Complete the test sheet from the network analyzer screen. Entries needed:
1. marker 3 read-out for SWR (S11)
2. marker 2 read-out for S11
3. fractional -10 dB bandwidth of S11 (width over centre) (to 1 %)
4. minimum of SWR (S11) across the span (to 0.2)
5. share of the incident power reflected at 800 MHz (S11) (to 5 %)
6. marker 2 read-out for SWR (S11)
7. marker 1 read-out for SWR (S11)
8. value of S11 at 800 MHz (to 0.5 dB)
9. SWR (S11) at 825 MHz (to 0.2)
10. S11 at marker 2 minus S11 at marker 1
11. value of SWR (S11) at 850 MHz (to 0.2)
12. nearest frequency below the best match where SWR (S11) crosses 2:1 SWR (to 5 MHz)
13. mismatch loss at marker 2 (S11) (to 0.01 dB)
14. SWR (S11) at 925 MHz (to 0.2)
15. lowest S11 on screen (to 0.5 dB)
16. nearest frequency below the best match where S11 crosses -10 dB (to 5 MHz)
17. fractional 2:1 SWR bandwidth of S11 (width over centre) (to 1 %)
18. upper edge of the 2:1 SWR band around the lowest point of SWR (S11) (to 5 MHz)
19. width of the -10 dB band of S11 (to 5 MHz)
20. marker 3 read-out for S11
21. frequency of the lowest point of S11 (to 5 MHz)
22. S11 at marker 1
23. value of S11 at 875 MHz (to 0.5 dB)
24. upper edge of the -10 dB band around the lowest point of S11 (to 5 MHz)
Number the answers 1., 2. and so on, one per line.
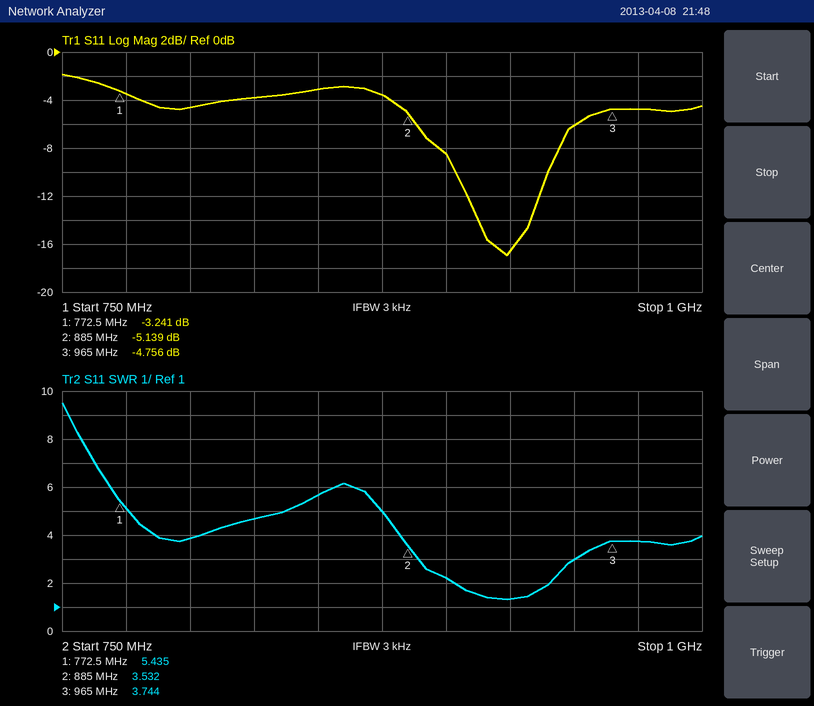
1. 3.744
2. -5.139 dB
3. 4 %
4. 1.4
5. 35 %
6. 3.532
7. 5.435
8. -4.5 dB
9. 4.6
10. -1.898 dB
11. 5.6
12. 905 MHz
13. 1.59 dB
14. 1.4
15. -17.0 dB
16. 905 MHz
17. 4 %
18. 940 MHz
19. 35 MHz
20. -4.756 dB
21. 925 MHz
22. -3.241 dB
23. -3.5 dB
24. 940 MHz
